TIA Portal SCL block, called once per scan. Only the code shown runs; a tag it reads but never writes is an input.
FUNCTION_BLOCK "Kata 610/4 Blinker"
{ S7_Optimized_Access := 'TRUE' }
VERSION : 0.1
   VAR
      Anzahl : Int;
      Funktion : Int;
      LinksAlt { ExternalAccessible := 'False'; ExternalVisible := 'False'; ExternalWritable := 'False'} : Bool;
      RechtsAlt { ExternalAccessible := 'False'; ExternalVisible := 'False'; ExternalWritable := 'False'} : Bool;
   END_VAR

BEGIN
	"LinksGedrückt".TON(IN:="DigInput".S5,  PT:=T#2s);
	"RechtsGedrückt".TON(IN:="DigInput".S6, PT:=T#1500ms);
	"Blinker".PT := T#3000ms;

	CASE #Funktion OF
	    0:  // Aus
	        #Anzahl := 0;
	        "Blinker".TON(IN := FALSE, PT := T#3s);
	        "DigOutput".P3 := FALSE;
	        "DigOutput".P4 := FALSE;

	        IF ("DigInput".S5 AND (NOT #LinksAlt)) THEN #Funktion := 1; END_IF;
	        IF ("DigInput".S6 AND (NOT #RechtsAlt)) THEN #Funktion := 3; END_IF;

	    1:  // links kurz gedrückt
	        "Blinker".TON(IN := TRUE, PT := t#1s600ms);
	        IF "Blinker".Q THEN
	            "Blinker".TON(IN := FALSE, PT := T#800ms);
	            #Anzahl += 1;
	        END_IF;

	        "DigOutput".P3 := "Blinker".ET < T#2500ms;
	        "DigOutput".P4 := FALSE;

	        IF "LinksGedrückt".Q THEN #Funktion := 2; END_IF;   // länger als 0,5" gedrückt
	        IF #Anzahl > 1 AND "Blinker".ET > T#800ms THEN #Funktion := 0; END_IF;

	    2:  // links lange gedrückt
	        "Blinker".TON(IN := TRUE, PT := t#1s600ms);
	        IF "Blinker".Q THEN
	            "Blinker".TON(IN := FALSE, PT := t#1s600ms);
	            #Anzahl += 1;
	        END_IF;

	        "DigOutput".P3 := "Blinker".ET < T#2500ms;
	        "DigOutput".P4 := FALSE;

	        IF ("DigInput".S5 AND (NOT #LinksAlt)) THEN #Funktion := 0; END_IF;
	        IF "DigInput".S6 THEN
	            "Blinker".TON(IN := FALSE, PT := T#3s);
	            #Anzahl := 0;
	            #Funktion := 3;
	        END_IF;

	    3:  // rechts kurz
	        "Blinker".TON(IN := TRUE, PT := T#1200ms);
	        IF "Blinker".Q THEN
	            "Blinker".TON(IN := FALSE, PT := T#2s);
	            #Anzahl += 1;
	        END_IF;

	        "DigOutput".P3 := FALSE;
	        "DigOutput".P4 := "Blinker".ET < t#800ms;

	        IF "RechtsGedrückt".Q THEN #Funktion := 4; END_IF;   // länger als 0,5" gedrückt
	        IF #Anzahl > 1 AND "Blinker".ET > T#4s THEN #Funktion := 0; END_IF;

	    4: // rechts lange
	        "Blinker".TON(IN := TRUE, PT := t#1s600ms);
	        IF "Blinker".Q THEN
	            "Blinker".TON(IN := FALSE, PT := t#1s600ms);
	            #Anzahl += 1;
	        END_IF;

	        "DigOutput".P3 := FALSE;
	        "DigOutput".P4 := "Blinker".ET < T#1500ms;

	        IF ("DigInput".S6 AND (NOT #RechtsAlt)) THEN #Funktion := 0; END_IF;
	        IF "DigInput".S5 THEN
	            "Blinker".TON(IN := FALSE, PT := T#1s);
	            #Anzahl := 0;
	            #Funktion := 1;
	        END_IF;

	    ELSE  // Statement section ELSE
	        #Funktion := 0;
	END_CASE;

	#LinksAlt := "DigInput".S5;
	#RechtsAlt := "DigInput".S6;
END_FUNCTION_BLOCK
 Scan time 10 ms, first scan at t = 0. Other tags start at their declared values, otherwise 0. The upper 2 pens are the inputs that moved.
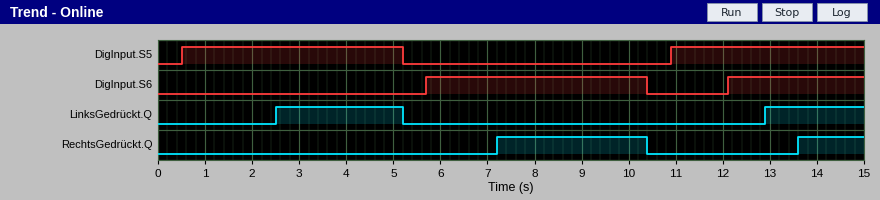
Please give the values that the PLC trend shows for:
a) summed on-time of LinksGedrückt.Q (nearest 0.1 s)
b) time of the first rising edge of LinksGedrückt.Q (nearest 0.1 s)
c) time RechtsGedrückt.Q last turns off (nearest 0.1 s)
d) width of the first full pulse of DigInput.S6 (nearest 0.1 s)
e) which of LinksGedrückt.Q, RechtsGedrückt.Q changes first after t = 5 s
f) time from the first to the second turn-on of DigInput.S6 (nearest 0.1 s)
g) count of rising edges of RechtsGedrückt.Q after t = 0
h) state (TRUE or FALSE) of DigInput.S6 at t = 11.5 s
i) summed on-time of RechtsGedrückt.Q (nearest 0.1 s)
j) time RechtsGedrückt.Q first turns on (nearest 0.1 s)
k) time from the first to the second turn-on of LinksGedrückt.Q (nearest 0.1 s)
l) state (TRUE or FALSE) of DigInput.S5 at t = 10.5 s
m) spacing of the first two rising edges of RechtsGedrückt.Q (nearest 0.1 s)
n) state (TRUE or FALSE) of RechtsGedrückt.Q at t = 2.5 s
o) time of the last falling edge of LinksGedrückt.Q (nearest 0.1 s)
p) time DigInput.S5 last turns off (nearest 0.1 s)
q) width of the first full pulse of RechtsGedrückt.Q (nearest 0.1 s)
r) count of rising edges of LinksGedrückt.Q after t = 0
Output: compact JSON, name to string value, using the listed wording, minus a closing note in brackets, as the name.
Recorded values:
{"summed on-time of LinksGedrückt.Q": "4.8 s", "time of the first rising edge of LinksGedrückt.Q": "2.5 s", "time RechtsGedrückt.Q last turns off": "10.4 s", "width of the first full pulse of DigInput.S6": "4.7 s", "which of LinksGedrückt.Q, RechtsGedrückt.Q changes first after t = 5 s": "LinksGedrückt.Q", "time from the first to the second turn-on of DigInput.S6": "6.4 s", "count of rising edges of RechtsGedrückt.Q after t = 0": "2", "state (TRUE or FALSE) of DigInput.S6 at t = 11.5 s": "FALSE", "summed on-time of RechtsGedrückt.Q": "4.6 s", "time RechtsGedrückt.Q first turns on": "7.2 s", "time from the first to the second turn-on of LinksGedrückt.Q": "10.4 s", "state (TRUE or FALSE) of DigInput.S5 at t = 10.5 s": "FALSE", "spacing of the first two rising edges of RechtsGedrückt.Q": "6.4 s", "state (TRUE or FALSE) of RechtsGedrückt.Q at t = 2.5 s": "FALSE", "time of the last falling edge of LinksGedrückt.Q": "5.2 s", "time DigInput.S5 last turns off": "5.2 s", "width of the first full pulse of RechtsGedrückt.Q": "3.2 s", "count of rising edges of LinksGedrückt.Q after t = 0": "2"}
